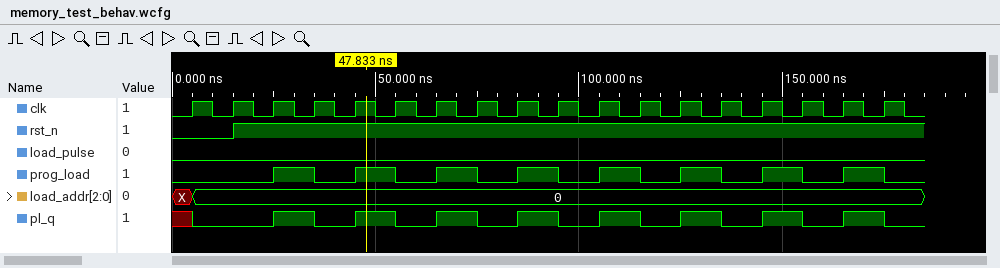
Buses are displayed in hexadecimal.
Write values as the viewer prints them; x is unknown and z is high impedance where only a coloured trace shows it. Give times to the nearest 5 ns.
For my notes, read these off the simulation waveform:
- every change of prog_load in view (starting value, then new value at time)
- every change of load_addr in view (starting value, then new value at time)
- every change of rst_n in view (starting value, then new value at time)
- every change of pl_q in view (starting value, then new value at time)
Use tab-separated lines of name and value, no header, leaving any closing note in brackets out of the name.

every change of prog_load in view	0, 1 at 25 ns, 0 at 35 ns, 1 at 45 ns, 0 at 55 ns, 1 at 65 ns, 0 at 75 ns, 1 at 85 ns, 0 at 95 ns, 1 at 105 ns, 0 at 115 ns, 1 at 125 ns, 0 at 135 ns, 1 at 145 ns, 0 at 155 ns, 1 at 165 ns, 0 at 175 ns
every change of load_addr in view	X, 0 at 5 ns
every change of rst_n in view	0, 1 at 15 ns
every change of pl_q in view	x, 0 at 5 ns, 1 at 25 ns, 0 at 35 ns, 1 at 45 ns, 0 at 55 ns, 1 at 65 ns, 0 at 75 ns, 1 at 85 ns, 0 at 95 ns, 1 at 105 ns, 0 at 115 ns, 1 at 125 ns, 0 at 135 ns, 1 at 145 ns, 0 at 155 ns, 1 at 165 ns, 0 at 175 ns
